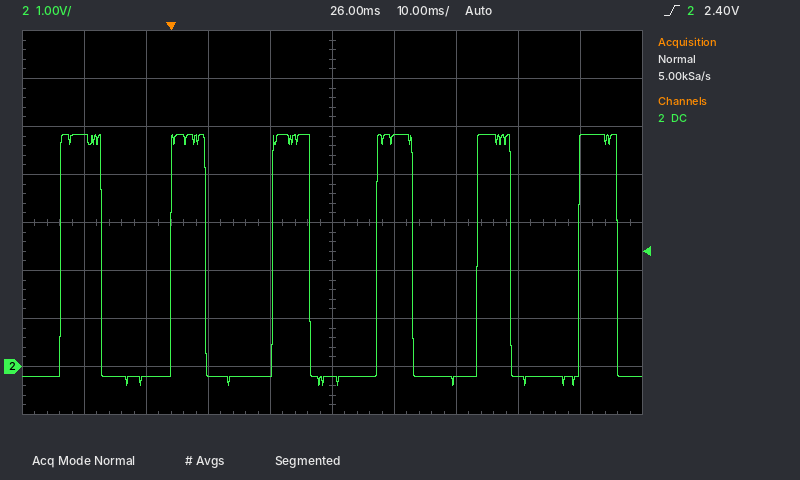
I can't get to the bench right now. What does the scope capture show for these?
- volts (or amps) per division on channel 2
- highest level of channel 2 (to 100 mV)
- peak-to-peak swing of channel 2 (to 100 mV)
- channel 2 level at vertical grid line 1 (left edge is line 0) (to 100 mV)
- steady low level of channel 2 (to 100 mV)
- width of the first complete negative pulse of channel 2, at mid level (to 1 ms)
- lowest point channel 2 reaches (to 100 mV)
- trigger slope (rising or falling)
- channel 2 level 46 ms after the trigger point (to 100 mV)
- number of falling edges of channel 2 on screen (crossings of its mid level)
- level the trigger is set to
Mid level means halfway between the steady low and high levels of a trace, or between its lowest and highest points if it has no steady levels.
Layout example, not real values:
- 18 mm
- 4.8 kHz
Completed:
- 1 V
- 4.8 V
- 5.2 V
- 4.8 V
- -200 mV
- 11 ms
- -400 mV
- rising
- -300 mV
- 6
- 2.40 V
